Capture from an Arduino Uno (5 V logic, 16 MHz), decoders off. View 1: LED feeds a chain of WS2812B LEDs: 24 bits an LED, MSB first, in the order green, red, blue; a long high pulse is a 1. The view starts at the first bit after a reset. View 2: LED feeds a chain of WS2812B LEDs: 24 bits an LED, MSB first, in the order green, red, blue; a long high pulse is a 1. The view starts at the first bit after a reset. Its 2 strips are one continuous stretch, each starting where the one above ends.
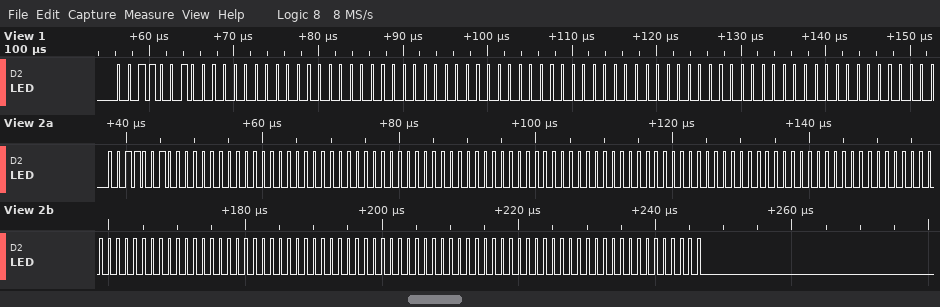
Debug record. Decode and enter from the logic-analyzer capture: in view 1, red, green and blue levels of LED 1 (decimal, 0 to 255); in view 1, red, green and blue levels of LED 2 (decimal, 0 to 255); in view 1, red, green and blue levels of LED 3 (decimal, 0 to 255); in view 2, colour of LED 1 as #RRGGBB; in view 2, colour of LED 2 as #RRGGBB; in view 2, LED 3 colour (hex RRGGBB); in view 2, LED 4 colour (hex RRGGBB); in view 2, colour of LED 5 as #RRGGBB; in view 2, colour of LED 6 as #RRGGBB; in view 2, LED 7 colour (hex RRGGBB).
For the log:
0, 50, 0
0, 0, 0
0, 0, 0
#003200
#000000
#000000
#000000
#000000
#000000
#000000
